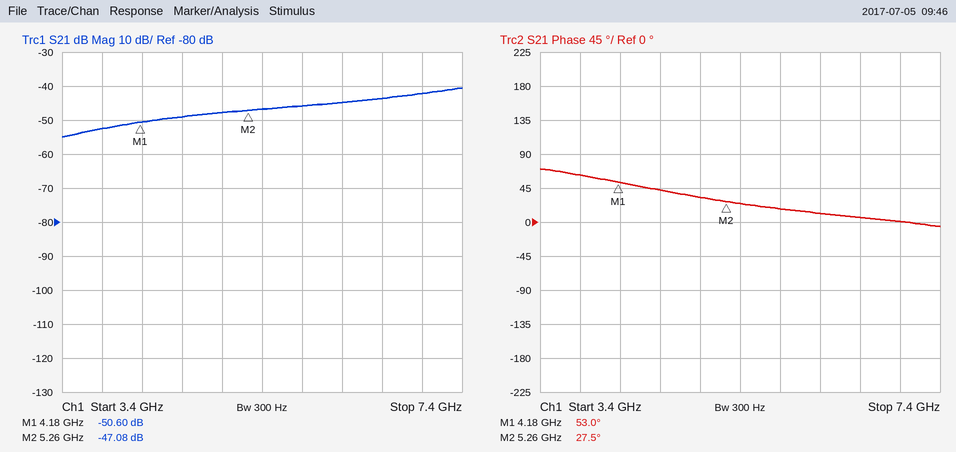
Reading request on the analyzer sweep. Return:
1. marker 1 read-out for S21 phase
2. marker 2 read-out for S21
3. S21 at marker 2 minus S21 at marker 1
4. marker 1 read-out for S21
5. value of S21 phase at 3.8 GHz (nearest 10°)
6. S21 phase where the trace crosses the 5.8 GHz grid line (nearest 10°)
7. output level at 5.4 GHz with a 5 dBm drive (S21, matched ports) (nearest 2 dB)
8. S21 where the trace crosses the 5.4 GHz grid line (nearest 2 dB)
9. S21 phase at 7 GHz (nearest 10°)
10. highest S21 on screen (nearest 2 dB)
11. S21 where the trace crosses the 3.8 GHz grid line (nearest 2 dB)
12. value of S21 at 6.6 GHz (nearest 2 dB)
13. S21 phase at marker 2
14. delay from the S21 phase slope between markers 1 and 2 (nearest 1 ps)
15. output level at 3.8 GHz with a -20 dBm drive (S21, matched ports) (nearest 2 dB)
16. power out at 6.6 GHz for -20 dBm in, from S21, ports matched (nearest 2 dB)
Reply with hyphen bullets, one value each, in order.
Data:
- 53.0°
- -47.08 dB
- 3.52 dB
- -50.60 dB
- 60°
- 20°
- -42 dBm
- -46 dB
- 0°
- -40 dB
- -52 dB
- -44 dB
- 27.5°
- 66 ps
- -72 dBm
- -64 dBm
